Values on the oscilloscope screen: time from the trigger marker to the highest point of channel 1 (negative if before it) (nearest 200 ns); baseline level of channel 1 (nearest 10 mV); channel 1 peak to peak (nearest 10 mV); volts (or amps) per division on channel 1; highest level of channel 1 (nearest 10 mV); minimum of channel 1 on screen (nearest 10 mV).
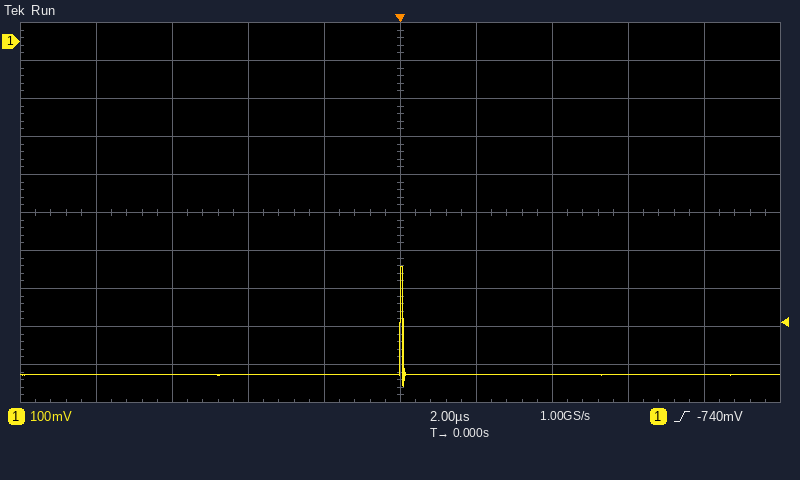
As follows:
0.0 µs
-880 mV
320 mV
100 mV
-590 mV
-910 mV
